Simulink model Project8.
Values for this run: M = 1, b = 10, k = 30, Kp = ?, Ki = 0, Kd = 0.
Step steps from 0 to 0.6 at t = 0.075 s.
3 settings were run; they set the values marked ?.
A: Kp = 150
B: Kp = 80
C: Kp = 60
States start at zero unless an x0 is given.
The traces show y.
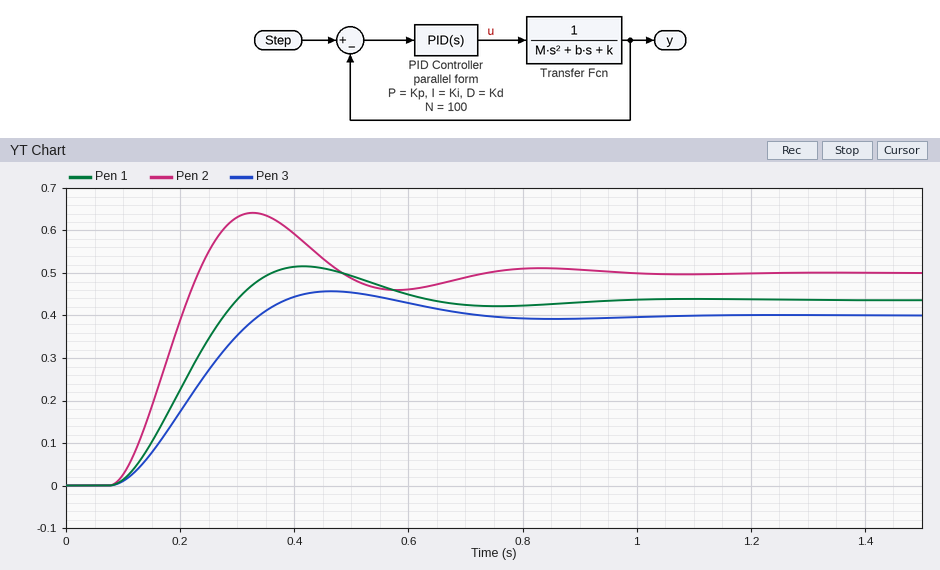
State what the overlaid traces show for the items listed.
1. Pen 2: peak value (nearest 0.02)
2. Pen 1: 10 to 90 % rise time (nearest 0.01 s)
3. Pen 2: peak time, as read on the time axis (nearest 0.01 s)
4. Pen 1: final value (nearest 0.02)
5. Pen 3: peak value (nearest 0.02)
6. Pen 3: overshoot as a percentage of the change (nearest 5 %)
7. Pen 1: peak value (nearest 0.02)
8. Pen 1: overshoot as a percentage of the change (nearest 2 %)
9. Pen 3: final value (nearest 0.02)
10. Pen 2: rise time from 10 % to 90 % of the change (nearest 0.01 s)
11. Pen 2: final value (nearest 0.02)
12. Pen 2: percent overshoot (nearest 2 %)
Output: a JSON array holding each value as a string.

["0.64", "0.15 s", "0.33 s", "0.44", "0.46", "15 %", "0.52", "18 %", "0.40", "0.11 s", "0.50", "28 %"]
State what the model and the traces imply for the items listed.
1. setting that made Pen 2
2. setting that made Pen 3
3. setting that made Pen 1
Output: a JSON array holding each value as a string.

["A", "C", "B"]
